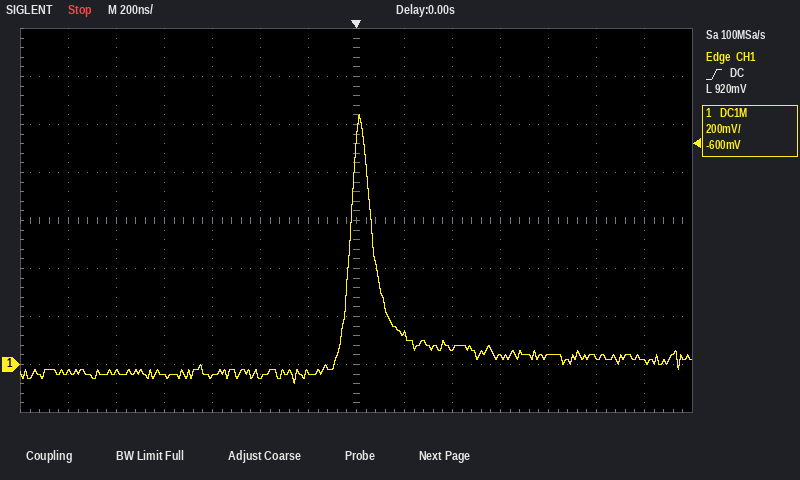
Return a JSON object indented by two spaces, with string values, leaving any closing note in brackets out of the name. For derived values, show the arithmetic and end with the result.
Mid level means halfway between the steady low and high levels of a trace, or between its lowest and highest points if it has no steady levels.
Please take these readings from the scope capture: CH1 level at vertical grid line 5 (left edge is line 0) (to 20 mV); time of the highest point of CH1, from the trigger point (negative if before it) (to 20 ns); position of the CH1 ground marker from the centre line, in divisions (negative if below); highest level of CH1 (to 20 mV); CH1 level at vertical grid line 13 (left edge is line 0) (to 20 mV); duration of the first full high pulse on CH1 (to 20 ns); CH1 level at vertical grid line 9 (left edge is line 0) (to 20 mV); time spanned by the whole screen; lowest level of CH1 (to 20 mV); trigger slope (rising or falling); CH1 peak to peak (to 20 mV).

{
  "CH1 level at vertical grid line 5 (left edge is line 0)": "-60 mV",
  "time of the highest point of CH1, from the trigger point (negative if before it)": "+20 ns",
  "position of the CH1 ground marker from the centre line, in divisions": "-3.0 div",
  "highest level of CH1": "1.04 V",
  "CH1 level at vertical grid line 13 (left edge is line 0)": "20 mV",
  "duration of the first full high pulse on CH1": "100 ns",
  "CH1 level at vertical grid line 9 (left edge is line 0)": "60 mV",
  "time spanned by the whole screen": "2.8 µs",
  "lowest level of CH1": "-80 mV",
  "trigger slope": "rising",
  "CH1 peak to peak": "1.04 V − (-80 mV) = 1.12 V"
}
